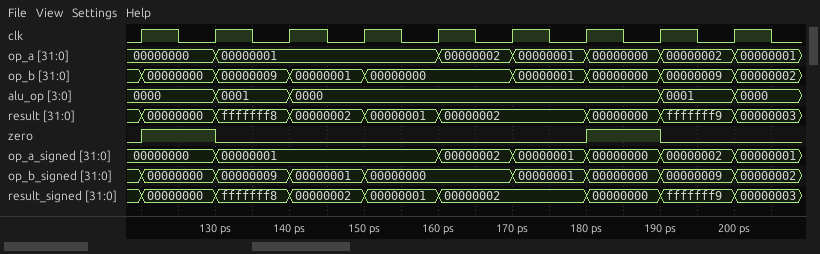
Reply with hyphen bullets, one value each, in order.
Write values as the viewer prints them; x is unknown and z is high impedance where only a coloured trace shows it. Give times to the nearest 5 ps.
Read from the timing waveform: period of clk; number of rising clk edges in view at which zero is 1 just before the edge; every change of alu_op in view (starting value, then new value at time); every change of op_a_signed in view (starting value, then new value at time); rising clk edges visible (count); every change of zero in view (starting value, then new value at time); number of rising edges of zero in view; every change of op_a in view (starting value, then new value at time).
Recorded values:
- 10 ps
- 2
- 0000, 0001 at 130 ps, 0000 at 140 ps, 0001 at 190 ps, 0000 at 200 ps
- 00000000, 00000001 at 130 ps, 00000002 at 160 ps, 00000001 at 170 ps, 00000000 at 180 ps, 00000002 at 190 ps, 00000001 at 200 ps
- 9
- 0, 1 at 120 ps, 0 at 130 ps, 1 at 180 ps, 0 at 190 ps
- 2
- 00000000, 00000001 at 130 ps, 00000002 at 160 ps, 00000001 at 170 ps, 00000000 at 180 ps, 00000002 at 190 ps, 00000001 at 200 ps
